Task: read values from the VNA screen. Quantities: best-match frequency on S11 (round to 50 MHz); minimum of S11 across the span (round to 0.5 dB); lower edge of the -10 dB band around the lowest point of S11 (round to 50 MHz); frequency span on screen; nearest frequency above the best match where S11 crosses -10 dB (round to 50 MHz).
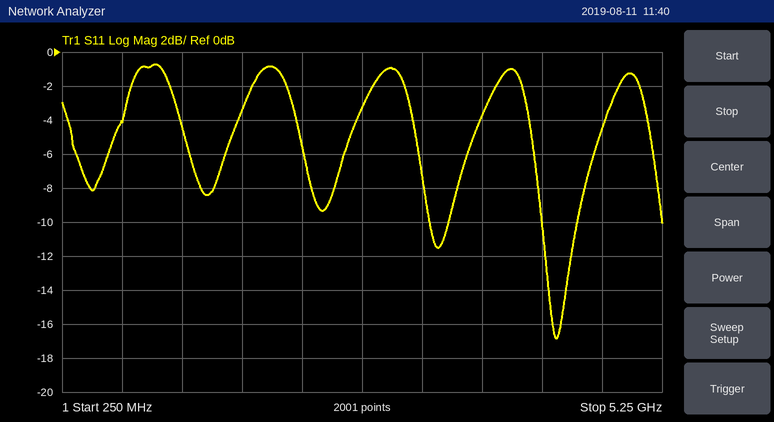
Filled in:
4.35 GHz
-17.0 dB
4.25 GHz
5 GHz
4.55 GHz
